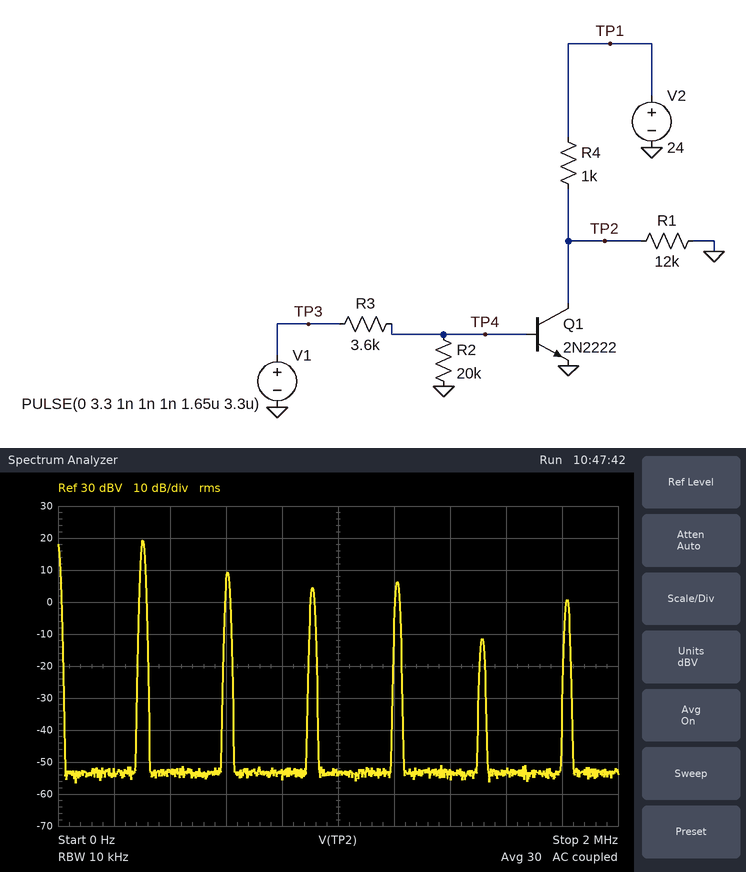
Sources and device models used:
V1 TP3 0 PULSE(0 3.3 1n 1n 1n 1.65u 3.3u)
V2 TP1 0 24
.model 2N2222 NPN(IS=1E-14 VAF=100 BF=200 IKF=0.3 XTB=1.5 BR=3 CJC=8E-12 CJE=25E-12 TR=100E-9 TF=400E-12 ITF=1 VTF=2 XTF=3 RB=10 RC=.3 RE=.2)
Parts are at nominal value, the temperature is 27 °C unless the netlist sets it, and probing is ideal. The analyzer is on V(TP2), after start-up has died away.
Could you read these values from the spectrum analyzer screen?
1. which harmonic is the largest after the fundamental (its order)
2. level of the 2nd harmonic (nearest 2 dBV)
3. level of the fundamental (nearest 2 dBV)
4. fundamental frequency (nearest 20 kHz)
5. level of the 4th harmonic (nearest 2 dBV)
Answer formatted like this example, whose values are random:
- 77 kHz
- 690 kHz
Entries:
- 2
- 10 dBV
- 20 dBV
- 300 kHz
- 6 dBV
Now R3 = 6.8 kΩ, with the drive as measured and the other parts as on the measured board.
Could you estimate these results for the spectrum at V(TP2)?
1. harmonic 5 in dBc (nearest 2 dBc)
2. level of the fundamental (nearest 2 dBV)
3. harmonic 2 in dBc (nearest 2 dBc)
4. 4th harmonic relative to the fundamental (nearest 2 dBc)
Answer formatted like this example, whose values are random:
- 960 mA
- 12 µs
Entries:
- -24 dBc
- 20 dBV
- -14 dBc
- -18 dBc
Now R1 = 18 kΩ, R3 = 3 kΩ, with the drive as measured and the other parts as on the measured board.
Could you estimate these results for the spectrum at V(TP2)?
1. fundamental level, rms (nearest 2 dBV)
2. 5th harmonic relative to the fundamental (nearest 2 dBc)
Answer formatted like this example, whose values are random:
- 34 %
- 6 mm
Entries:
- 20 dBV
- -28 dBc
